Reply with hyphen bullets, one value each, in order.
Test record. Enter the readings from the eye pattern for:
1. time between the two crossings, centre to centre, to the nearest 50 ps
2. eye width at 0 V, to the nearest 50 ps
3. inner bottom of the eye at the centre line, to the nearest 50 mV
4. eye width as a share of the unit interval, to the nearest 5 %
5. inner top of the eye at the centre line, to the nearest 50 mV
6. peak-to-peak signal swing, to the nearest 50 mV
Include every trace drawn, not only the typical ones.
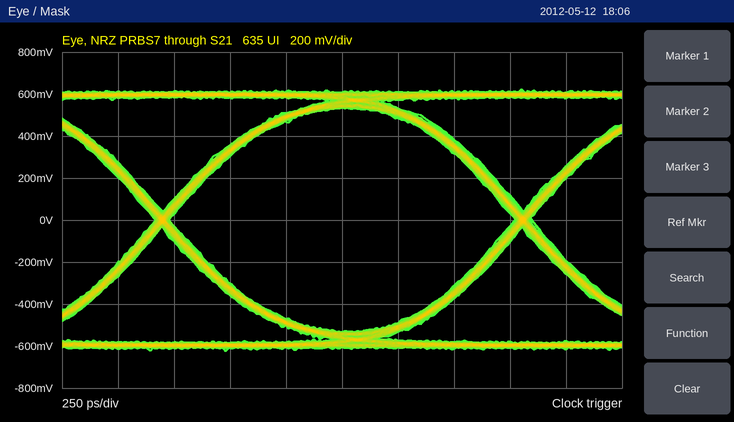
- 1.60 ns
- 1.55 ns
- -550 mV
- 95 %
- 550 mV
- 1.25 V
